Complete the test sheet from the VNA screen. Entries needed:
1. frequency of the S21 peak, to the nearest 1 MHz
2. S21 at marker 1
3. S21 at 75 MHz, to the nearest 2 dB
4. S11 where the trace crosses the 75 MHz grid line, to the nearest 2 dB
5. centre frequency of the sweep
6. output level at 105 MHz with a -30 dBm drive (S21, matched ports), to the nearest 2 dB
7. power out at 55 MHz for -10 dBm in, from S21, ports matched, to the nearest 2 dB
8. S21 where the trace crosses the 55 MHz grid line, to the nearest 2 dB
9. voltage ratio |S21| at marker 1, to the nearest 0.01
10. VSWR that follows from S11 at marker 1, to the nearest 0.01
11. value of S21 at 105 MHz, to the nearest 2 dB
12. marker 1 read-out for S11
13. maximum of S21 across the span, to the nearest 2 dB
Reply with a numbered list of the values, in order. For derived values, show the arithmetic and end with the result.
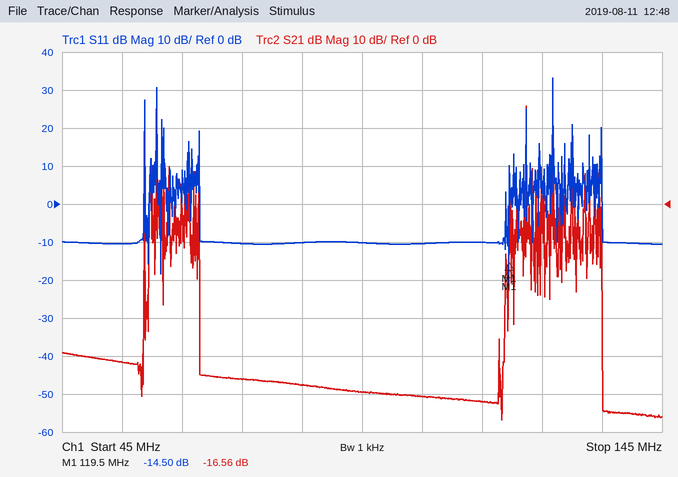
1. 122 MHz
2. -16.56 dB
3. -46 dB
4. -10 dB
5. 95 MHz
6. -30 dBm + (-50 dB) = -80 dBm
7. -10 dBm + (-42 dB) = -52 dBm
8. -42 dB
9. 10^(-16.56/20) ≈ 0.15
10. (1 + 0.1884)/(1 − 0.1884) ≈ 1.46
11. -50 dB
12. -14.50 dB
13. 26 dB
